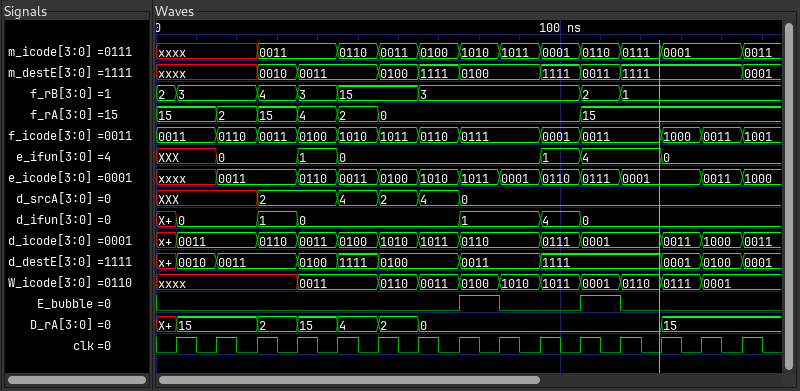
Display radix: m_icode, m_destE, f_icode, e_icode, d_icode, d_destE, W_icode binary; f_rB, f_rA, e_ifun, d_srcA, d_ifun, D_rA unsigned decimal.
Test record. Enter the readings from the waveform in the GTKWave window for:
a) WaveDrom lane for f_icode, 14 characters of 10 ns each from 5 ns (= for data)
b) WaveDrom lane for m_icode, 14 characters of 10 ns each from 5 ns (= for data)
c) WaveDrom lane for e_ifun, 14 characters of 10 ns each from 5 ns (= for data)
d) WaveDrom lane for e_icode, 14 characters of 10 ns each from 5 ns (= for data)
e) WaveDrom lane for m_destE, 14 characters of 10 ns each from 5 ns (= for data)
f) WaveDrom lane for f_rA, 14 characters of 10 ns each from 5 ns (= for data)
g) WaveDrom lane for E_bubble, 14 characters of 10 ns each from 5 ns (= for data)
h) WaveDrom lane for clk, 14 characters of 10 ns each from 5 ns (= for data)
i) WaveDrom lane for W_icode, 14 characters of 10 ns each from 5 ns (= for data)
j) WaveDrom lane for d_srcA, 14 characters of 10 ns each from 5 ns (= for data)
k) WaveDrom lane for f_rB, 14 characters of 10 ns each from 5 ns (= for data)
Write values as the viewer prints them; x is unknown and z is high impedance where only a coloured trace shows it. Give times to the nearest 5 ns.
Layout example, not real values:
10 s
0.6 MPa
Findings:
{name: 'f_icode', wave: '========.==.==', data: '0011 0110 0011 0100 1010 1011 0110 0111 0001 0011 1000 0011'}
{name: 'm_icode', wave: 'x.=.=========.', data: '0011 0110 0011 0100 1010 1011 0001 0110 0111 0001'}
{name: 'e_ifun', wave: 'x=.==....==.=.', data: '0 1 0 1 4 0'}
{name: 'e_icode', wave: 'x=.=========.=', data: '0011 0110 0011 0100 1010 1011 0001 0110 0111 0001 0011'}
{name: 'm_destE', wave: 'x.==.===.===..', data: '0010 0011 0100 1111 0100 1111 0011 1111'}
{name: 'f_rA', wave: '======....=...', data: '15 2 15 4 2 0 15'}
{name: 'E_bubble', wave: '0......10.10..'}
{name: 'clk', wave: 'p.............'}
{name: 'W_icode', wave: 'x..=.=========', data: '0011 0110 0011 0100 1010 1011 0001 0110 0111 0001'}
{name: 'd_srcA', wave: 'x.=.====......', data: '2 4 2 4 0'}
{name: 'f_rB', wave: '=.===.=...==..', data: '3 4 3 15 3 2 1'}
